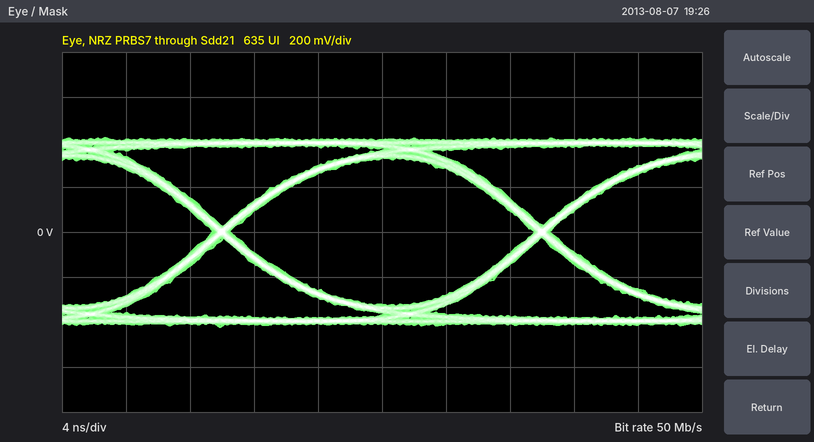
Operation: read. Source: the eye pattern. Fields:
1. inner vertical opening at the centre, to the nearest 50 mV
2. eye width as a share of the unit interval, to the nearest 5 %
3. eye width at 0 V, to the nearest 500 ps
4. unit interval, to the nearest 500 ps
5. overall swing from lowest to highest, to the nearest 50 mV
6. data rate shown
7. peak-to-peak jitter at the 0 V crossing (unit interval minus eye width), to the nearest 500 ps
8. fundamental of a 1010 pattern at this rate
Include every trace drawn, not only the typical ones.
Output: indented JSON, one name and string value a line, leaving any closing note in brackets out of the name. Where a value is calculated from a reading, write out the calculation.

{
  "inner vertical opening at the centre, to the nearest 50 mV": "650 mV",
  "eye width as a share of the unit interval, to the nearest 5 %": "19.0 ns / 20.0 ns ≈ 95 %",
  "eye width at 0 V, to the nearest 500 ps": "19.0 ns",
  "unit interval, to the nearest 500 ps": "20.0 ns",
  "overall swing from lowest to highest, to the nearest 50 mV": "850 mV",
  "data rate shown": "50 Mb/s",
  "peak-to-peak jitter at the 0 V crossing (unit interval minus eye width), to the nearest 500 ps": "1.0 ns",
  "fundamental of a 1010 pattern at this rate": "25 MHz"
}
